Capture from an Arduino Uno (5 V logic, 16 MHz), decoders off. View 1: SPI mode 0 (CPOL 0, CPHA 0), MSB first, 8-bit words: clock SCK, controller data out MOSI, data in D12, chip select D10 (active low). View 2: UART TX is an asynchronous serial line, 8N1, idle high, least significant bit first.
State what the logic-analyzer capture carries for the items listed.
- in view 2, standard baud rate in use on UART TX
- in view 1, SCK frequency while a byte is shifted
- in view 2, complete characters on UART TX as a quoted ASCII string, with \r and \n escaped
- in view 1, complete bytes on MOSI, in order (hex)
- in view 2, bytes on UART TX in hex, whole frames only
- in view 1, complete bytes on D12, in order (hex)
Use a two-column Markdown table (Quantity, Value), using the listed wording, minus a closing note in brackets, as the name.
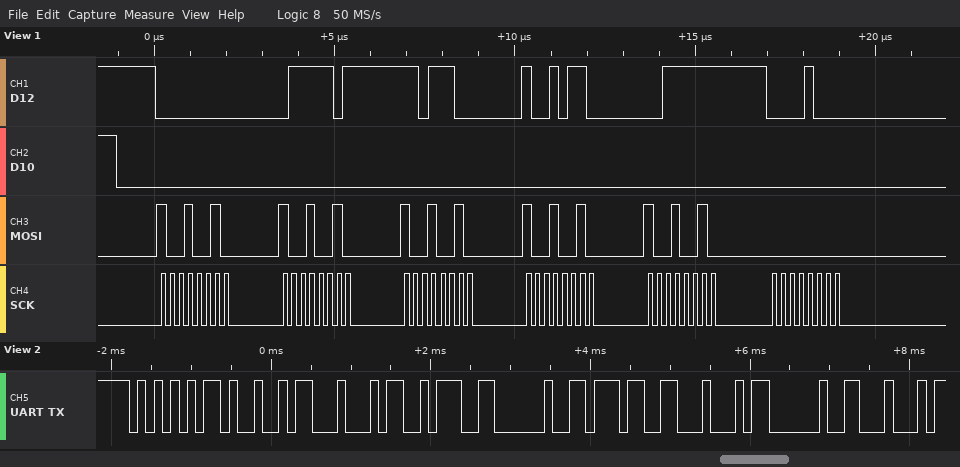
| Quantity | Value |
|---|---|
| in view 2, standard baud rate in use on UART TX | 9600 baud |
| in view 1, SCK frequency while a byte is shifted | 4 MHz |
| in view 2, complete characters on UART TX as a quoted ASCII string, with \r and \n escaped | "UID: 7D D" |
| in view 1, complete bytes on MOSI, in order | 92 92 92 92 92 00 |
| in view 2, bytes on UART TX in hex, whole frames only | 55 49 44 3A 20 37 44 20 44 |
| in view 1, complete bytes on D12, in order | 00 7D DC 96 3F 08 |
